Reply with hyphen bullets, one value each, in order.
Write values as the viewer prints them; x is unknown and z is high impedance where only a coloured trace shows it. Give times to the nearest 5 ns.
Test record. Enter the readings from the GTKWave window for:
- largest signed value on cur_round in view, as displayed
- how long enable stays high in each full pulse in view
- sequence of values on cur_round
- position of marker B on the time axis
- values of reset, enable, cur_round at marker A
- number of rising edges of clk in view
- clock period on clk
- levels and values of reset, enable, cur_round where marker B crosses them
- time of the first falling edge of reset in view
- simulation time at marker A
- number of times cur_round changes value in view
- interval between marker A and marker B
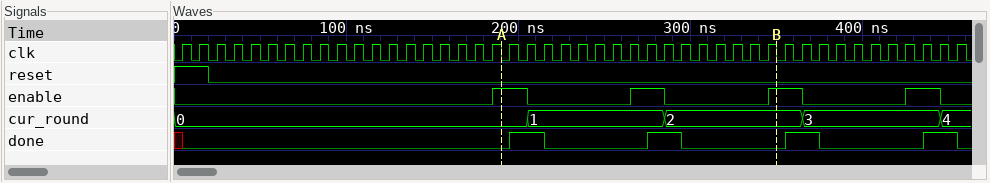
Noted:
- 4
- 20 ns, 20 ns, 20 ns, 20 ns
- 0, 1, 2, 3, 4
- 350 ns
- reset=0, enable=1, cur_round=0
- 46
- 10 ns
- reset=0, enable=1, cur_round=2
- 20 ns
- 190 ns
- 4
- 160 ns
